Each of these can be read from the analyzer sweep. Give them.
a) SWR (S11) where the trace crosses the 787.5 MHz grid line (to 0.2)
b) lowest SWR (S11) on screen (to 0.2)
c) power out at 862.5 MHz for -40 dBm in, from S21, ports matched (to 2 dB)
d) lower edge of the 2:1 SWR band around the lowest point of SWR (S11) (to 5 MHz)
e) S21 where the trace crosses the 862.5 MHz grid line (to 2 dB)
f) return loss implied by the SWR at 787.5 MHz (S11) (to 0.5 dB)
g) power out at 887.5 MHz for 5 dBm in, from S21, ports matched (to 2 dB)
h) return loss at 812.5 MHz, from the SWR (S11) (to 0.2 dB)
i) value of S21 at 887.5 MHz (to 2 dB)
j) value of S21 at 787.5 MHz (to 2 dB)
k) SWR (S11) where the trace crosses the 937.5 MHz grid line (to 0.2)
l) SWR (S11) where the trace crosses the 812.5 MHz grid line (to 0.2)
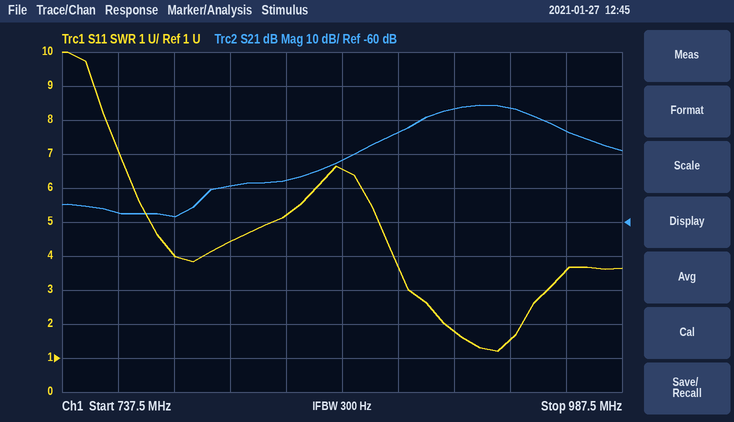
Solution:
4.0
1.2
-82 dBm
910 MHz
-42 dB
4.5 dB
-28 dBm
4.0 dB
-34 dB
-58 dB
1.6
4.4
